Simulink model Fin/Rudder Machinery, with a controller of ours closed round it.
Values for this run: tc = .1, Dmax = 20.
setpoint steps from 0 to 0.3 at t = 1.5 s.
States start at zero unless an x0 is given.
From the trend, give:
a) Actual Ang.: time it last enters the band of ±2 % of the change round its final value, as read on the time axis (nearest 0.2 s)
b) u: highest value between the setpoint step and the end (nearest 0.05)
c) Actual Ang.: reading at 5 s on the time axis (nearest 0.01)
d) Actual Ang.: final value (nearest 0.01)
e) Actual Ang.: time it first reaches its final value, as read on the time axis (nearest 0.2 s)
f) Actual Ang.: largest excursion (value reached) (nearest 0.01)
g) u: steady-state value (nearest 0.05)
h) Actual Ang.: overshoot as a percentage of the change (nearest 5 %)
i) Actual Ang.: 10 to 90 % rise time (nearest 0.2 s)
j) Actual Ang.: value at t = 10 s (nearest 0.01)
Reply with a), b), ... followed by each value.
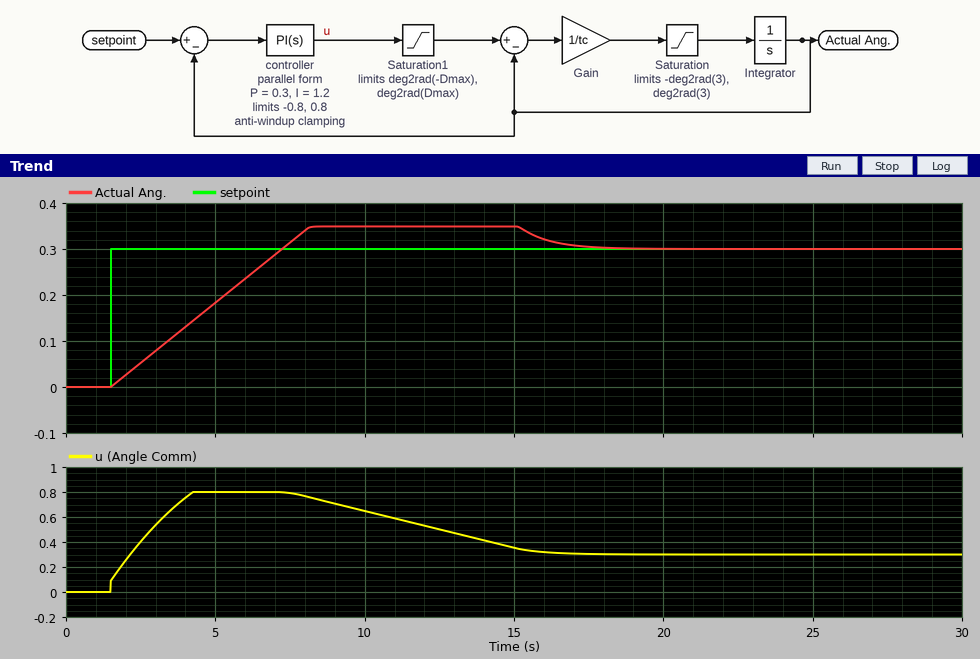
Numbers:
a) 17.2 s
b) 0.80
c) 0.18
d) 0.30
e) 7.2 s
f) 0.35
g) 0.30
h) 15 %
i) 4.6 s
j) 0.35
